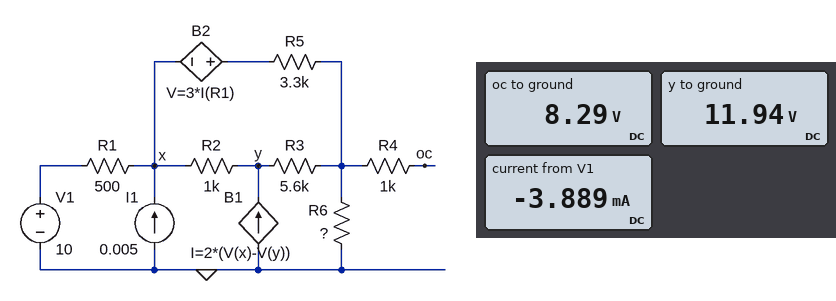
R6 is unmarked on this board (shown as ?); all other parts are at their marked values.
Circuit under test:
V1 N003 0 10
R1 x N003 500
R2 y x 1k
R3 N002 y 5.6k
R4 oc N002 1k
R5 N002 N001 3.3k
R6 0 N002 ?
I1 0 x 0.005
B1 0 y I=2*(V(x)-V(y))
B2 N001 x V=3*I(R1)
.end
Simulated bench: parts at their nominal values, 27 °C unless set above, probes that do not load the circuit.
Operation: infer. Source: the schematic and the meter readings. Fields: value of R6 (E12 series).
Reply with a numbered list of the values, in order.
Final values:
1. 4.7 kΩ
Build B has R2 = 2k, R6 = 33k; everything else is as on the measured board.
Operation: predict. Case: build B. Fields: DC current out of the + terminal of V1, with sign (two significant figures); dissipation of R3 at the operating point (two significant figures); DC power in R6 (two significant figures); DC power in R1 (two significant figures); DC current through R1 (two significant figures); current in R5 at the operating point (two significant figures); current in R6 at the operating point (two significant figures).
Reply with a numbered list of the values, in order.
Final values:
1. -4.8 mA
2. 94 µW
3. 4.1 mW
4. 11 mW
5. 4.8 mA
6. 220 µA
7. 350 µA
